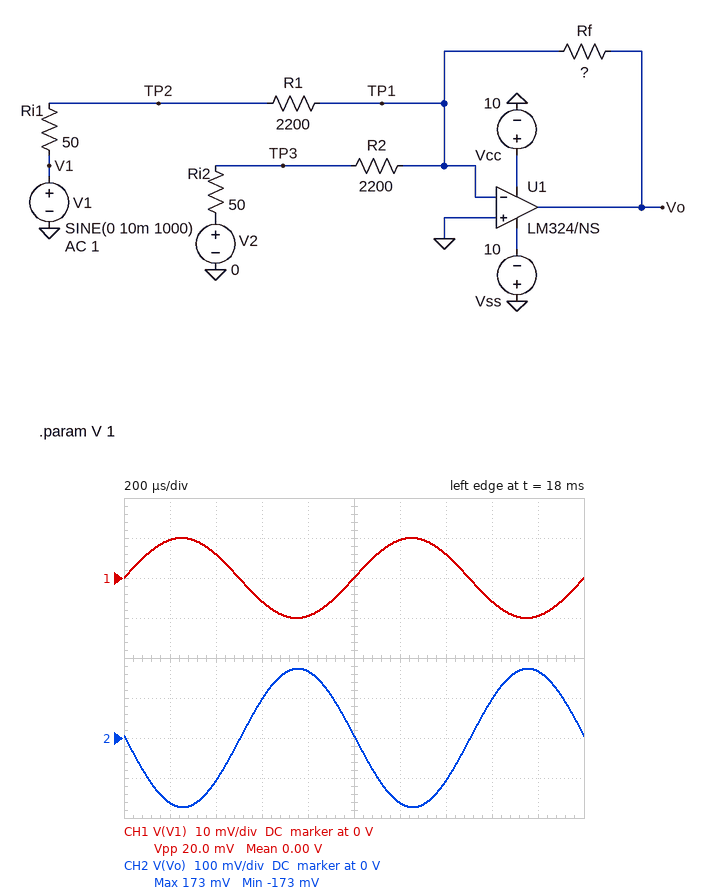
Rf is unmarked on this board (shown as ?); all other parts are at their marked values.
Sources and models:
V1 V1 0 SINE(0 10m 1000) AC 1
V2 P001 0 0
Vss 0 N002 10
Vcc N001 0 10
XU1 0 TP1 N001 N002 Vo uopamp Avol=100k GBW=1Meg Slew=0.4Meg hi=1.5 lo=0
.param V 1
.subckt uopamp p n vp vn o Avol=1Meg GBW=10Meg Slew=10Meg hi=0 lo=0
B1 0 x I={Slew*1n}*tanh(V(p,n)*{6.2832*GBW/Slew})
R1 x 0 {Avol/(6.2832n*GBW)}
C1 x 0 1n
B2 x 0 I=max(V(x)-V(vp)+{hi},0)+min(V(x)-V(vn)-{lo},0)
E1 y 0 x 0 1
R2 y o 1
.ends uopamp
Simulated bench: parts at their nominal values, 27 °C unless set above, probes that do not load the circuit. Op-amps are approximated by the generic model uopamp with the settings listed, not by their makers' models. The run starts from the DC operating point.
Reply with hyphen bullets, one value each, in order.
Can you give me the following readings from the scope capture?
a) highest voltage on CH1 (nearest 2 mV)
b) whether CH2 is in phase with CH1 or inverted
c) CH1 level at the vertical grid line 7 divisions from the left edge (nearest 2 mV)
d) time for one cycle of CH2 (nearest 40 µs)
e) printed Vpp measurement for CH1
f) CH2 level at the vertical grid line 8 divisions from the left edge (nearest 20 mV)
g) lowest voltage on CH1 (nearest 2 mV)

- 10 mV
- inverted
- 6 mV
- 1.00 ms
- 20.0 mV
- 100 mV
- -10 mV
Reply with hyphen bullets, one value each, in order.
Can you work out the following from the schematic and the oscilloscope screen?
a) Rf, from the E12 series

- 39 kΩ
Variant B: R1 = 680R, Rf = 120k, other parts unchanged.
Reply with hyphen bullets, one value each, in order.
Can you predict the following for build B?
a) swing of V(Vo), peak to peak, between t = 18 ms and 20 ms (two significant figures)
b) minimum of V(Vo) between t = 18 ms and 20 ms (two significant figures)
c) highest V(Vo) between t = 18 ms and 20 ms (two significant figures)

- 3.2 V
- -1.6 V
- 1.6 V
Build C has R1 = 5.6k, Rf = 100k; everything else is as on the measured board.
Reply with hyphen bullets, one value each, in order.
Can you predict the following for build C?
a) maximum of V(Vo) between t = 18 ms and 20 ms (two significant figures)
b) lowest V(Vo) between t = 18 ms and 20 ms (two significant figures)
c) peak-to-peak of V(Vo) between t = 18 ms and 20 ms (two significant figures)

- 180 mV
- -180 mV
- 350 mV
